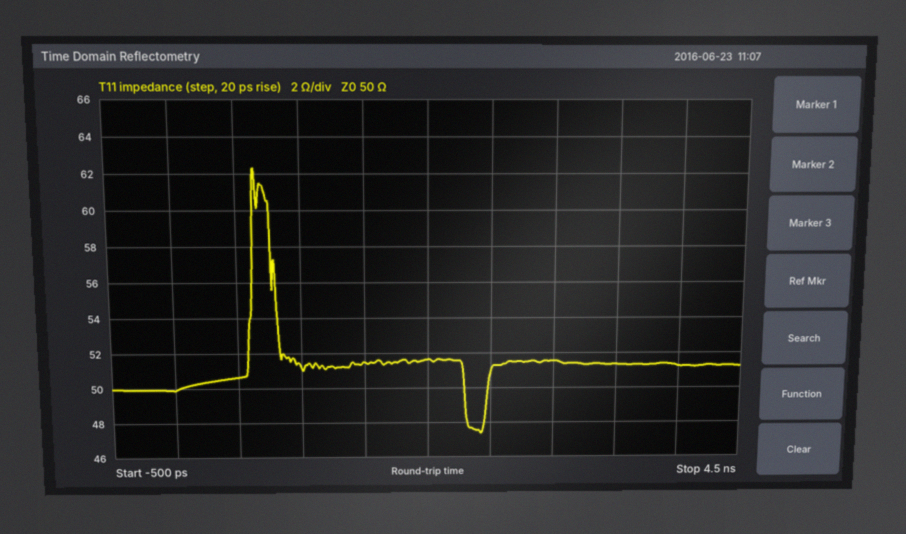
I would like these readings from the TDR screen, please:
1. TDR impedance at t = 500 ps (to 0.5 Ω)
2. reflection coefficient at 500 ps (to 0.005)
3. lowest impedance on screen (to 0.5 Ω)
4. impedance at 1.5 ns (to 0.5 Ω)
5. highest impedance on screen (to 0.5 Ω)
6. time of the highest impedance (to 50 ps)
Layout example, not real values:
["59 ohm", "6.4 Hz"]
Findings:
["50.5 Ω", "+0.005", "47.5 Ω", "51.5 Ω", "62.5 Ω", "650 ps"]
